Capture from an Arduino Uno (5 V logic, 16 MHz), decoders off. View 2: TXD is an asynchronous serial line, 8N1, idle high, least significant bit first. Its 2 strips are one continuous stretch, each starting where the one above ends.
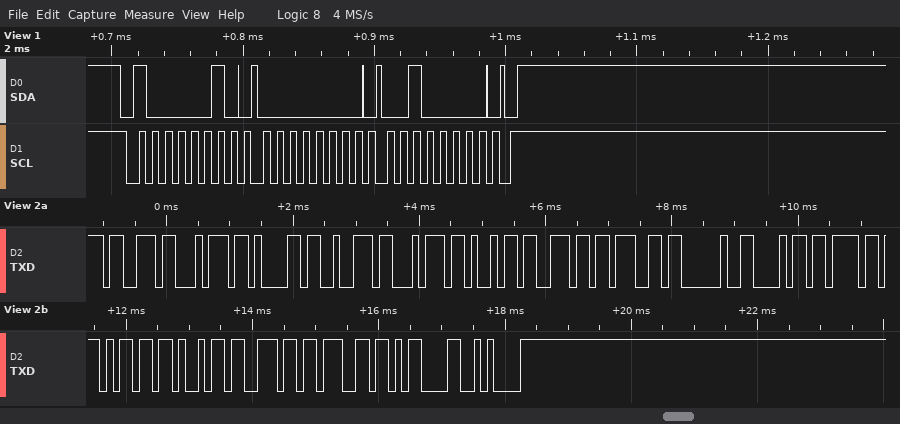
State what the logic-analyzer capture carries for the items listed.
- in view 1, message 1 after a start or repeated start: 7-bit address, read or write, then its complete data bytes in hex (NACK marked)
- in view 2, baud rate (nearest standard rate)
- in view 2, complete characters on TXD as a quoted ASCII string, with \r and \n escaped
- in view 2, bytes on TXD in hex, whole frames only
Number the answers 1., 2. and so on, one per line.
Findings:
1. 0x41 write: 00 20
2. 9600 baud
3. "starting homing\r\n"
4. 73 74 61 72 74 69 6E 67 20 68 6F 6D 69 6E 67 0D 0A
